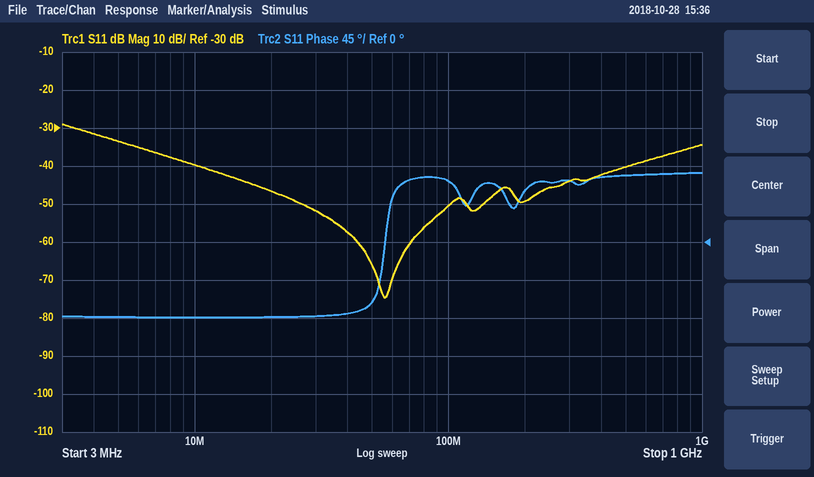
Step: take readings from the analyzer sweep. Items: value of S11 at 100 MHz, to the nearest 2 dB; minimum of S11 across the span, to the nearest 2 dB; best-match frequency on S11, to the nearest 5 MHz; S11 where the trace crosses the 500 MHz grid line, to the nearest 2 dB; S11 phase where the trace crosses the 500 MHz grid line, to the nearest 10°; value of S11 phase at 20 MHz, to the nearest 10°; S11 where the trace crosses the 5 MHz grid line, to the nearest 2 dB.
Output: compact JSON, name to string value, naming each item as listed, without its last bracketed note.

{"value of S11 at 100 MHz, to the nearest 2 dB": "-50 dB", "minimum of S11 across the span, to the nearest 2 dB": "-74 dB", "best-match frequency on S11, to the nearest 5 MHz": "55 MHz", "S11 where the trace crosses the 500 MHz grid line, to the nearest 2 dB": "-40 dB", "S11 phase where the trace crosses the 500 MHz grid line, to the nearest 10°": "80°", "value of S11 phase at 20 MHz, to the nearest 10°": "-90°", "S11 where the trace crosses the 5 MHz grid line, to the nearest 2 dB": "-34 dB"}
